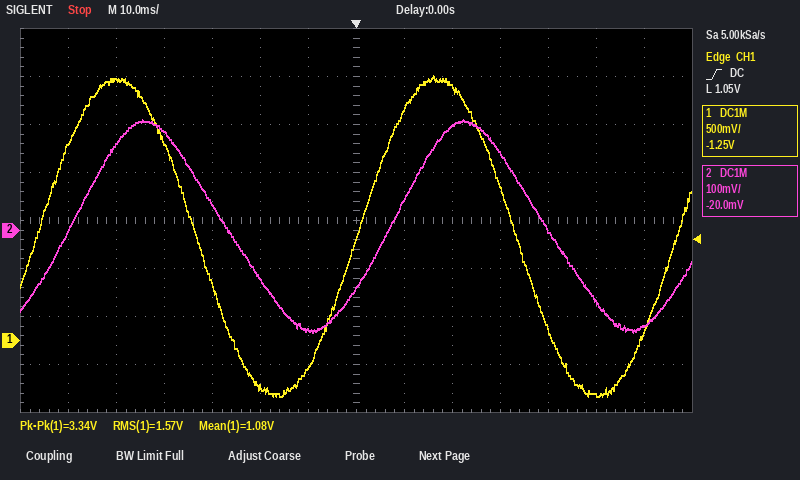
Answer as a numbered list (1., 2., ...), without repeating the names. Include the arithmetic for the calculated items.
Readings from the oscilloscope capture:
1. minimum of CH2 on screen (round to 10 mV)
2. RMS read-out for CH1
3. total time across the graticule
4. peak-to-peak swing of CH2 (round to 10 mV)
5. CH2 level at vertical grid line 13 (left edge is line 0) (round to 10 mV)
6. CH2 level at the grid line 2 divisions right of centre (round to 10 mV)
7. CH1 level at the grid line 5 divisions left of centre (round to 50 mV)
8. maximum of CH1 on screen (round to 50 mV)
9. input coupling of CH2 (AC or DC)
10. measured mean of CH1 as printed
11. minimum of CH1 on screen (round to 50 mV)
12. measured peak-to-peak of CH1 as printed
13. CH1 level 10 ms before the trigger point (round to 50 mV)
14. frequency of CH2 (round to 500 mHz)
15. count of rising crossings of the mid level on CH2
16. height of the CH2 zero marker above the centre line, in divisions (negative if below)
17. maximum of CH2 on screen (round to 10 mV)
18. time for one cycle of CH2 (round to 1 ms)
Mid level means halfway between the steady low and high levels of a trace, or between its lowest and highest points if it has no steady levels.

1. -210 mV
2. 1.57 V
3. 140 ms
4. 230 mV − (-210 mV) = 440 mV
5. -200 mV
6. 220 mV
7. 2.70 V
8. 2.75 V
9. DC
10. 1.08 V
11. -600 mV
12. 3.34 V
13. -300 mV
14. 1 / 67 ms ≈ 14.9 Hz, so 15.0 Hz to the nearest 500 mHz
15. 2
16. -0.2 div
17. 230 mV
18. 67 ms
